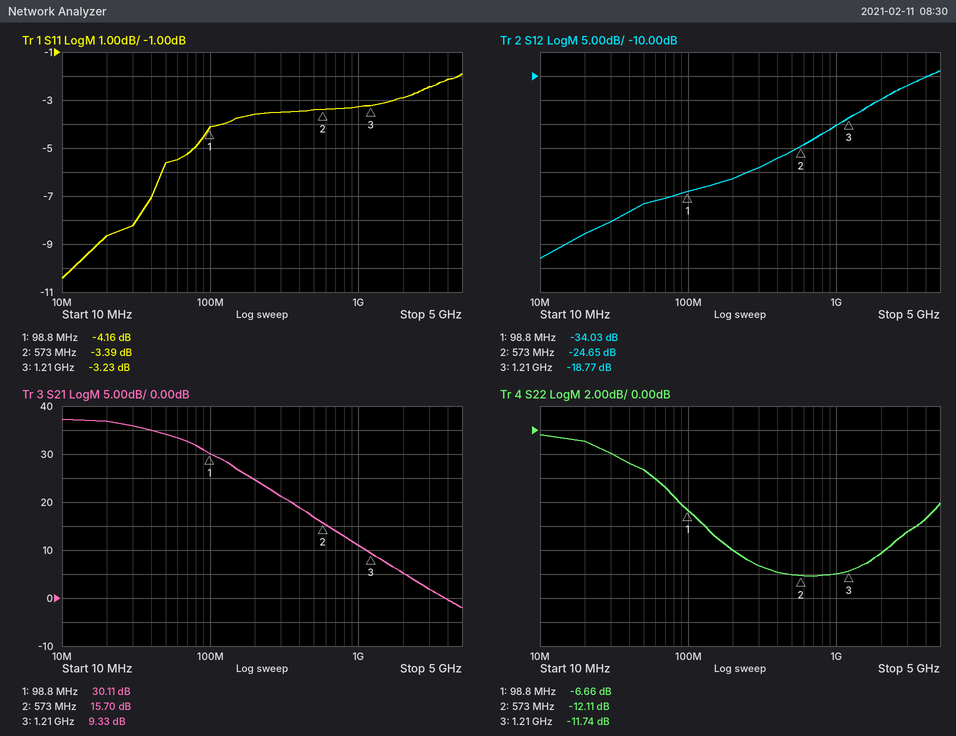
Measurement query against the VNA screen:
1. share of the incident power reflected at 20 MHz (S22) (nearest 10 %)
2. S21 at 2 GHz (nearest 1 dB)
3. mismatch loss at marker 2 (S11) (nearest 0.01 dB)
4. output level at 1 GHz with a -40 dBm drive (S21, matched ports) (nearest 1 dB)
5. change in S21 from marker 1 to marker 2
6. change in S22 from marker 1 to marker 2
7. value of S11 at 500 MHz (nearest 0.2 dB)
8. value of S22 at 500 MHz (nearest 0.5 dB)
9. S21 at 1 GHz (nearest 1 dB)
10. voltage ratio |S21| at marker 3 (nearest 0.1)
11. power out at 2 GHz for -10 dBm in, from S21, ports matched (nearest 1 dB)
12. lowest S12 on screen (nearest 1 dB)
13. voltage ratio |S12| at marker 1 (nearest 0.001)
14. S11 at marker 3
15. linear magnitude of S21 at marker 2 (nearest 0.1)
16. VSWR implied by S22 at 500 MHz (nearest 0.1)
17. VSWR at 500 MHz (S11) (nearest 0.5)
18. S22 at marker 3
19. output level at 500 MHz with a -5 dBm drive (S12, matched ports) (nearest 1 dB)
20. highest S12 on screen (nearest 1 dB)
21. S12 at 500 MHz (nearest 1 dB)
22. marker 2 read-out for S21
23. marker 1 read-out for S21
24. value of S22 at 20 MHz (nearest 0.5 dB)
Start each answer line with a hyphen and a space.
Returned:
- 80 %
- 5 dB
- 2.66 dB
- -29 dBm
- -14.41 dB
- -5.45 dB
- -3.4 dB
- -12.0 dB
- 11 dB
- 2.9
- -5 dBm
- -48 dB
- 0.020
- -3.23 dB
- 6.1
- 1.7
- 5.0
- -11.74 dB
- -31 dBm
- -9 dB
- -26 dB
- 15.70 dB
- 30.11 dB
- -1.0 dB
